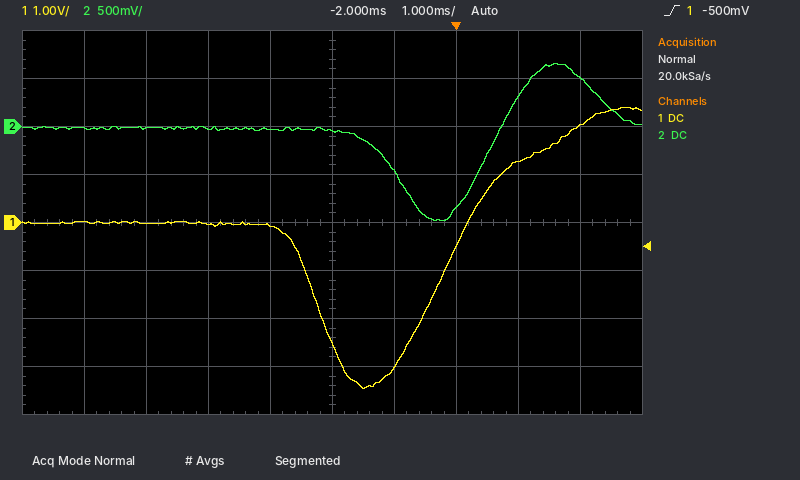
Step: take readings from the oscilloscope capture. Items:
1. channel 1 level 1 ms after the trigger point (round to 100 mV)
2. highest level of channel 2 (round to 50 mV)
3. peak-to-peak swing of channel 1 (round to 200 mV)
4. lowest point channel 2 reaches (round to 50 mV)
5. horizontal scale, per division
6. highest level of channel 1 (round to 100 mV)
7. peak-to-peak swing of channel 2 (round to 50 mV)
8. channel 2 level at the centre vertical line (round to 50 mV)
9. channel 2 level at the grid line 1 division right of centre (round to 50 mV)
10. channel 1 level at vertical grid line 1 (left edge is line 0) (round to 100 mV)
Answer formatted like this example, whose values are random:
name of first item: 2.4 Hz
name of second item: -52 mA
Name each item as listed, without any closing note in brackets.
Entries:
channel 1 level 1 ms after the trigger point: 1.3 V
highest level of channel 2: 650 mV
peak-to-peak swing of channel 1: 5.8 V
lowest point channel 2 reaches: -1.00 V
horizontal scale, per division: 1 ms
highest level of channel 1: 2.4 V
peak-to-peak swing of channel 2: 1.65 V
channel 2 level at the centre vertical line: -50 mV
channel 2 level at the grid line 1 division right of centre: -450 mV
channel 1 level at vertical grid line 1 (left edge is line 0): 0.0 V
